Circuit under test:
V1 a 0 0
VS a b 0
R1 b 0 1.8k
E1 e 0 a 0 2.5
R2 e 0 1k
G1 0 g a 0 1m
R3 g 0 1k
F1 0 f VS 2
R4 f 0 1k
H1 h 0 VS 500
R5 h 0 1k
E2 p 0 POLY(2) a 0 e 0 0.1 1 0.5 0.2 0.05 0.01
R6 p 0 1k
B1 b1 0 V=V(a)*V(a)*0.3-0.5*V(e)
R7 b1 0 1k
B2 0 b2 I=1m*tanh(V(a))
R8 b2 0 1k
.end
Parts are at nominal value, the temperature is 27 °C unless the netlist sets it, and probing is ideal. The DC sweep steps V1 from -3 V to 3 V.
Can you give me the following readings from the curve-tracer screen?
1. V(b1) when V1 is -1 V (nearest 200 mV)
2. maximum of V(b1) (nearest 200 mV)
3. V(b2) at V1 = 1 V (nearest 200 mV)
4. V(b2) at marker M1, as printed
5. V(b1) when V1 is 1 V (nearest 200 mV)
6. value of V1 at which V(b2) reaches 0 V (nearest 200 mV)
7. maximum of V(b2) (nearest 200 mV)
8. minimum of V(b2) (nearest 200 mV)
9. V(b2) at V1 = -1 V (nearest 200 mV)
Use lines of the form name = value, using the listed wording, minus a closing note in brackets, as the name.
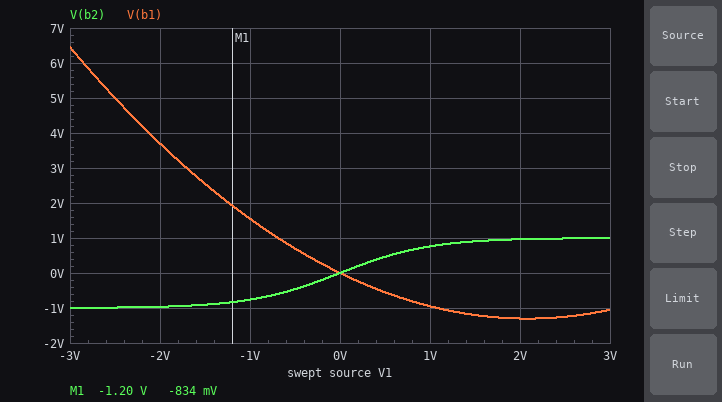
V(b1) when V1 is -1 V = 1.6 V
maximum of V(b1) = 6.4 V
V(b2) at V1 = 1 V = 800 mV
V(b2) at marker M1, as printed = -834 mV
V(b1) when V1 is 1 V = -1.0 V
value of V1 at which V(b2) reaches 0 V = 0 V
maximum of V(b2) = 1.0 V
minimum of V(b2) = -1.0 V
V(b2) at V1 = -1 V = -800 mV
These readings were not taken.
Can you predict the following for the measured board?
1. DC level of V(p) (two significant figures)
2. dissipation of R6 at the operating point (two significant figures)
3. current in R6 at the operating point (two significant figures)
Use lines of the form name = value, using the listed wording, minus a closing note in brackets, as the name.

DC level of V(p) = 100 mV
dissipation of R6 at the operating point = 10 µW
current in R6 at the operating point = 100 µA
